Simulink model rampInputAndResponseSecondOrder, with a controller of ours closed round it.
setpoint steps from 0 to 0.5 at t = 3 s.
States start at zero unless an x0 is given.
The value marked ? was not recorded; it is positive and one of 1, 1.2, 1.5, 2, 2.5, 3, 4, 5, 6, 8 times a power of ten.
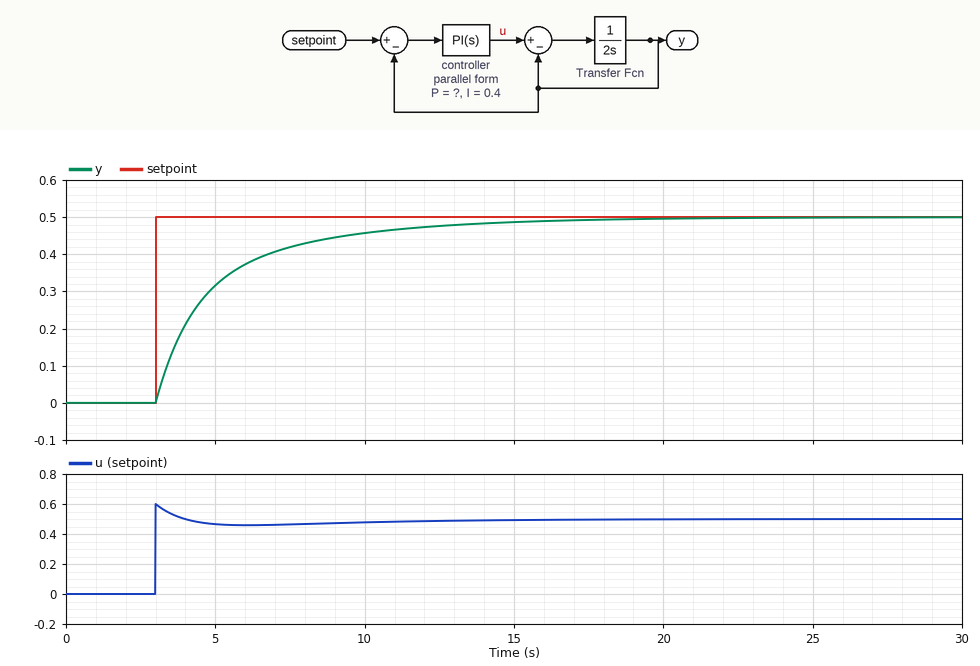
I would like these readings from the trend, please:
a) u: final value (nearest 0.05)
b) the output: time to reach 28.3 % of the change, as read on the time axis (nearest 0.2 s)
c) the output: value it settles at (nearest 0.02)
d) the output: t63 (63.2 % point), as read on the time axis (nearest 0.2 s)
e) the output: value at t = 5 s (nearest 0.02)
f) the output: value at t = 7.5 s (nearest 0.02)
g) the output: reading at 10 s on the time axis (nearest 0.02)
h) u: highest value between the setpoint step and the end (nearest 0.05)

0.50
3.6 s
0.50
5.0 s
0.32
0.42
0.46
0.60
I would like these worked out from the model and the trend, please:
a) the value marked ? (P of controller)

1.2
